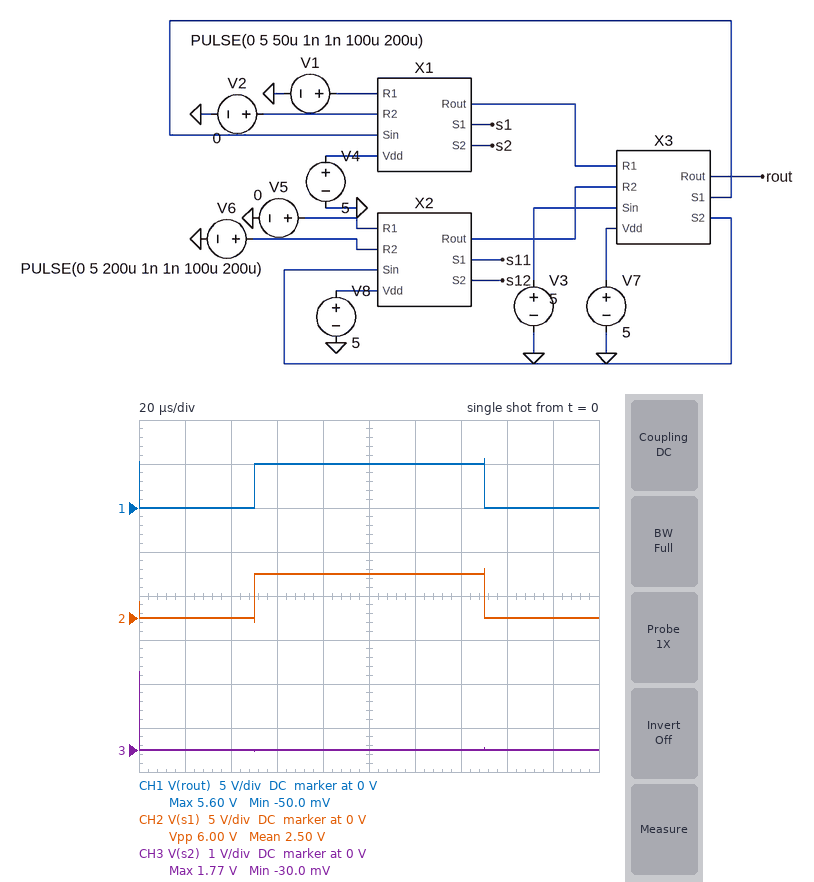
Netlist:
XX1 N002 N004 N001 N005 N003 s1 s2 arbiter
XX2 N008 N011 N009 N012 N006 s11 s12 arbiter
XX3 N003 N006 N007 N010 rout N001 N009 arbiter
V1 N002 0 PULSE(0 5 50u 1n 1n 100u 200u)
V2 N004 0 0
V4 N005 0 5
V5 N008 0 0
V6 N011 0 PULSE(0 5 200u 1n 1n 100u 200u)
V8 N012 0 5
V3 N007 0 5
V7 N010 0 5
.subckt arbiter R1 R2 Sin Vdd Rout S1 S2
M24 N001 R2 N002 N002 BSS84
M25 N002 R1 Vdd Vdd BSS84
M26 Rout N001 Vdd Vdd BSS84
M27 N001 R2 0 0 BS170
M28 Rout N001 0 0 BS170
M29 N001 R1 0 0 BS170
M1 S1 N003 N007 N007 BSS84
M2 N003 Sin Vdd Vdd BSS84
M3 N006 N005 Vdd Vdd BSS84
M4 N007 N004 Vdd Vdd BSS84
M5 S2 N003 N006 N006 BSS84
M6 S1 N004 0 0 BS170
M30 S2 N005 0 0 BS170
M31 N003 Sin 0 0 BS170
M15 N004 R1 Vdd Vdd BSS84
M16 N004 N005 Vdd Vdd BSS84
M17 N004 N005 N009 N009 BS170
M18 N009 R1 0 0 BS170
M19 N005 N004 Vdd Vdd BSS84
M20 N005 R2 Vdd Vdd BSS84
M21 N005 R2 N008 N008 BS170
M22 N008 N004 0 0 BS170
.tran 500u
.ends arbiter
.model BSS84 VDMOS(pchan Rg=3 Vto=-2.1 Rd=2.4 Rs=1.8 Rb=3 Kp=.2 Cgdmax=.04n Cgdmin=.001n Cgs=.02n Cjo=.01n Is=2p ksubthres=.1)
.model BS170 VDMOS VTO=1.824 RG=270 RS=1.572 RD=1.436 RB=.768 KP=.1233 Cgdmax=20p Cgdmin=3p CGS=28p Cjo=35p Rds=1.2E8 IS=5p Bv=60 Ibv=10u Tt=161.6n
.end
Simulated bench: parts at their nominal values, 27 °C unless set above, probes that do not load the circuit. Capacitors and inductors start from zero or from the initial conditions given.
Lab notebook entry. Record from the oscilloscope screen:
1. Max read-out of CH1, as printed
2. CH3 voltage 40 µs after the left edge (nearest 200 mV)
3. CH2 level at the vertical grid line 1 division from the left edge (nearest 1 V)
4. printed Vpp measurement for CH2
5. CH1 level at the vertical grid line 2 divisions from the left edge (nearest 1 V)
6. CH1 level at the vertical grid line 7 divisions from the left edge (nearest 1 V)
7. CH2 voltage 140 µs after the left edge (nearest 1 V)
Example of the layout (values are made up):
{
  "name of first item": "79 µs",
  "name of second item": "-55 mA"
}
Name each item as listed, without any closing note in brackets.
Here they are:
{
  "Max read-out of CH1, as printed": "5.60 V",
  "CH3 voltage 40 µs after the left edge": "0 V",
  "CH2 level at the vertical grid line 1 division from the left edge": "0 V",
  "printed Vpp measurement for CH2": "6.00 V",
  "CH1 level at the vertical grid line 2 divisions from the left edge": "0 V",
  "CH1 level at the vertical grid line 7 divisions from the left edge": "5 V",
  "CH2 voltage 140 µs after the left edge": "5 V"
}
